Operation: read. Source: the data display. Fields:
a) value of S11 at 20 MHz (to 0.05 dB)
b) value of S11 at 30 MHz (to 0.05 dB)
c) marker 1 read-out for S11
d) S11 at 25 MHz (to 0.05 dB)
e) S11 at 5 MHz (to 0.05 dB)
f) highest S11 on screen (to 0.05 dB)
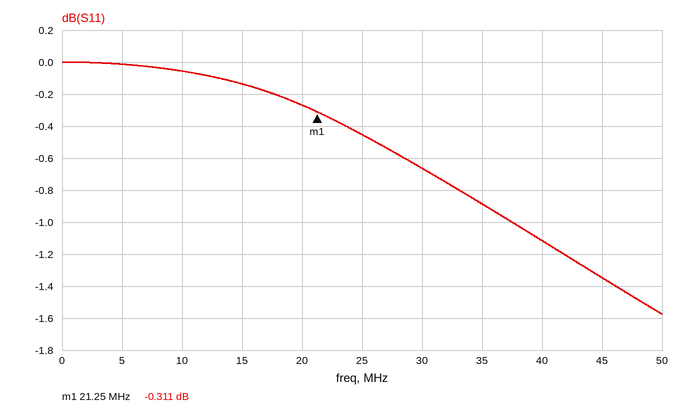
-0.25 dB
-0.65 dB
-0.311 dB
-0.45 dB
0.00 dB
0.00 dB
